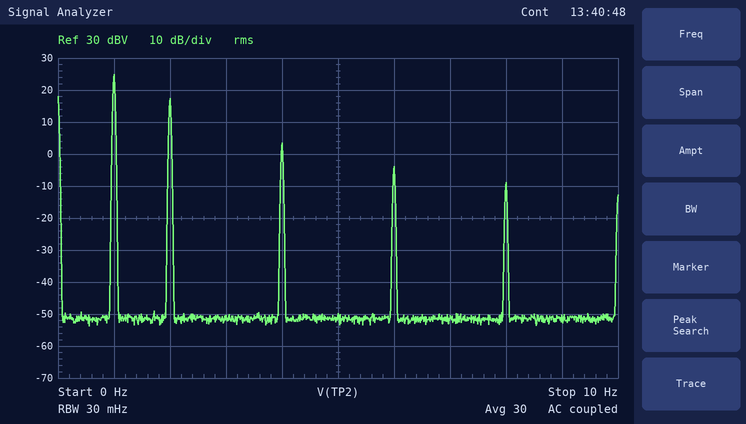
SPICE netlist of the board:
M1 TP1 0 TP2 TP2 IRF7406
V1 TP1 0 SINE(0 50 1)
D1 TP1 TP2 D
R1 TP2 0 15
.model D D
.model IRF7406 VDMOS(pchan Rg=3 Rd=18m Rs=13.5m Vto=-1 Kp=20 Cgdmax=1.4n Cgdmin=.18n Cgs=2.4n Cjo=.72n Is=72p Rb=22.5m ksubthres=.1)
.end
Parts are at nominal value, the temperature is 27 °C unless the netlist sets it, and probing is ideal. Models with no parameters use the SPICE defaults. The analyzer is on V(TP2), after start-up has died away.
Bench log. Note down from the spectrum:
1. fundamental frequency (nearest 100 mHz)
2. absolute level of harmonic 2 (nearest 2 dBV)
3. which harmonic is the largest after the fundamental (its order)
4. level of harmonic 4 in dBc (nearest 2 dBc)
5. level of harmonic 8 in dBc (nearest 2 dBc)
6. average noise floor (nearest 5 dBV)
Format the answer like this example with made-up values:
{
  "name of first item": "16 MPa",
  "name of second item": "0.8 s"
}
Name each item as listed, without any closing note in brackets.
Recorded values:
{
  "fundamental frequency": "1.0 Hz",
  "absolute level of harmonic 2": "18 dBV",
  "which harmonic is the largest after the fundamental": "2",
  "level of harmonic 4 in dBc": "-22 dBc",
  "level of harmonic 8 in dBc": "-34 dBc",
  "average noise floor": "-50 dBV"
}
